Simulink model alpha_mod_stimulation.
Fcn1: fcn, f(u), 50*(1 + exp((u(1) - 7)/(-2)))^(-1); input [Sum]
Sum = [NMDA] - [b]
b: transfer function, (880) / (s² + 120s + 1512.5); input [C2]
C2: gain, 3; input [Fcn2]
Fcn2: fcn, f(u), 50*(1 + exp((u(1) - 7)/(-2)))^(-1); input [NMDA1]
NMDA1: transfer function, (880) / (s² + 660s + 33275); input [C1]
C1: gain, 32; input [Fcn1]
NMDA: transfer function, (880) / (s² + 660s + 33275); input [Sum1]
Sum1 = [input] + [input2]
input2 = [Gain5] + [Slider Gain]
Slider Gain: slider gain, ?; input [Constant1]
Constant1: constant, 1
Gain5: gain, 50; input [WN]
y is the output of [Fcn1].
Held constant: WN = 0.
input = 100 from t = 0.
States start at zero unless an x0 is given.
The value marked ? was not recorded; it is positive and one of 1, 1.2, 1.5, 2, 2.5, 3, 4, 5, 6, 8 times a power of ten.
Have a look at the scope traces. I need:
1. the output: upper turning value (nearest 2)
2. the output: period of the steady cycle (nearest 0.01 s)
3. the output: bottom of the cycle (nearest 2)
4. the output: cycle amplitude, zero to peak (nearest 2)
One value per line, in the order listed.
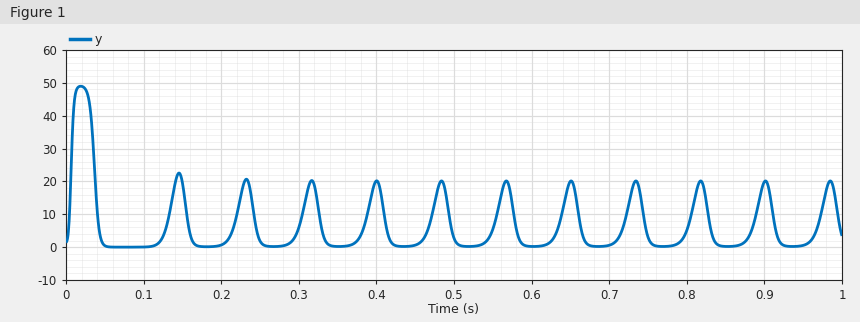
20
0.08 s
0
10
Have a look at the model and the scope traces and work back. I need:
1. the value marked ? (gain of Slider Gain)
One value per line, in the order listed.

1000
